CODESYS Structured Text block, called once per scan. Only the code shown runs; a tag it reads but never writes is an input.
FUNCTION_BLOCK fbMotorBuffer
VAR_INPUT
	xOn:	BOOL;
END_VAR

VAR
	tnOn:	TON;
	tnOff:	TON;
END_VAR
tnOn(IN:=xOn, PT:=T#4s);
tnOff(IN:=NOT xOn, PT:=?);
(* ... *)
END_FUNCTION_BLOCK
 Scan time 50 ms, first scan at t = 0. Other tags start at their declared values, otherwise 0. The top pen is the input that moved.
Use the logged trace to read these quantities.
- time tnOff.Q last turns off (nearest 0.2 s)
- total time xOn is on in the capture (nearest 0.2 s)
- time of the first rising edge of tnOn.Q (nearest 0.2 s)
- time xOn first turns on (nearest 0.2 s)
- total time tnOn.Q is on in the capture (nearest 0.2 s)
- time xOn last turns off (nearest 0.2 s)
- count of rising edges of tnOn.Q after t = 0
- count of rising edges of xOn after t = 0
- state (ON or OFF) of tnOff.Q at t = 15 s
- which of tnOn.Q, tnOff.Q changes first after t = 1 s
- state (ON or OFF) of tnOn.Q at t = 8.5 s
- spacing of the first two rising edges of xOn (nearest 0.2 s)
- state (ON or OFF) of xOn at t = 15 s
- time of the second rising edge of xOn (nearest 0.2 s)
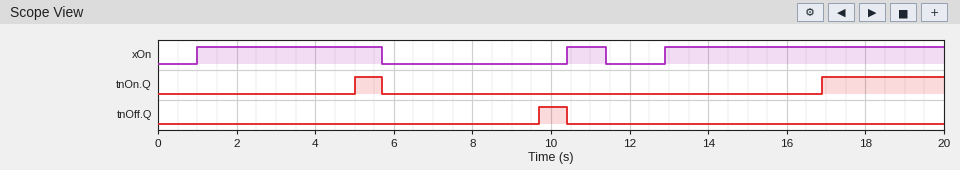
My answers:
10.4 s
12.8 s
5.0 s
1.0 s
3.8 s
11.4 s
2
3
OFF
tnOn.Q
OFF
9.4 s
ON
10.4 s
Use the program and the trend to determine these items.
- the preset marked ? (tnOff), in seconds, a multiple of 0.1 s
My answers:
4.0 s
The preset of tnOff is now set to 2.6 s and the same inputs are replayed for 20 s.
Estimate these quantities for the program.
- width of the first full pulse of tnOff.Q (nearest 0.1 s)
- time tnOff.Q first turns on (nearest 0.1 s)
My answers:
2.1 s
8.3 s
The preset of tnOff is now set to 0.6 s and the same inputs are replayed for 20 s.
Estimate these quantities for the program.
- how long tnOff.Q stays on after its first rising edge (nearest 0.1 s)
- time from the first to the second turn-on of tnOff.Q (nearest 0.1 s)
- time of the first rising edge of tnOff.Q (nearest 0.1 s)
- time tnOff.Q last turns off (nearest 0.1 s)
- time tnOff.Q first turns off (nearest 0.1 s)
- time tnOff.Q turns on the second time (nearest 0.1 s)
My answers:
0.4 s
5.7 s
0.6 s
12.9 s
1.0 s
6.3 s
